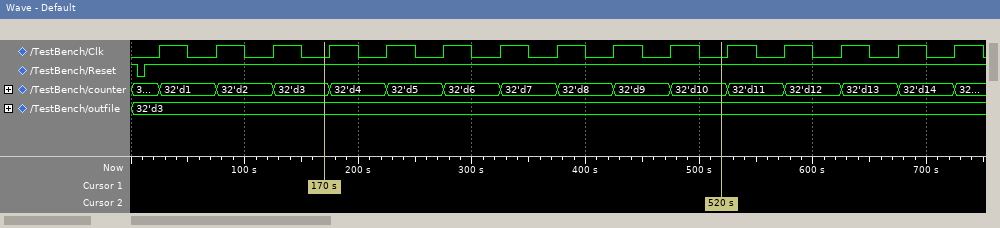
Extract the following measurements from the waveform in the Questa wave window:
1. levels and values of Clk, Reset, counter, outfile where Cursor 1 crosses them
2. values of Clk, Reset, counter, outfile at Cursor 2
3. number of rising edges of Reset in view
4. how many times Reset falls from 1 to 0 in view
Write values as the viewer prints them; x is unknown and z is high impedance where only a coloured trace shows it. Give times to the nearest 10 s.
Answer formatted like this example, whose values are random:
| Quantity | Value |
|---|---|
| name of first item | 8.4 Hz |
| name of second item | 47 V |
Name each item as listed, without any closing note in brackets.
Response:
| Quantity | Value |
|---|---|
| levels and values of Clk, Reset, counter, outfile where Cursor 1 crosses them | Clk=0, Reset=1, counter=32'd3, outfile=32'd3 |
| values of Clk, Reset, counter, outfile at Cursor 2 | Clk=0, Reset=1, counter=32'd10, outfile=32'd3 |
| number of rising edges of Reset in view | 1 |
| how many times Reset falls from 1 to 0 in view | 1 |
